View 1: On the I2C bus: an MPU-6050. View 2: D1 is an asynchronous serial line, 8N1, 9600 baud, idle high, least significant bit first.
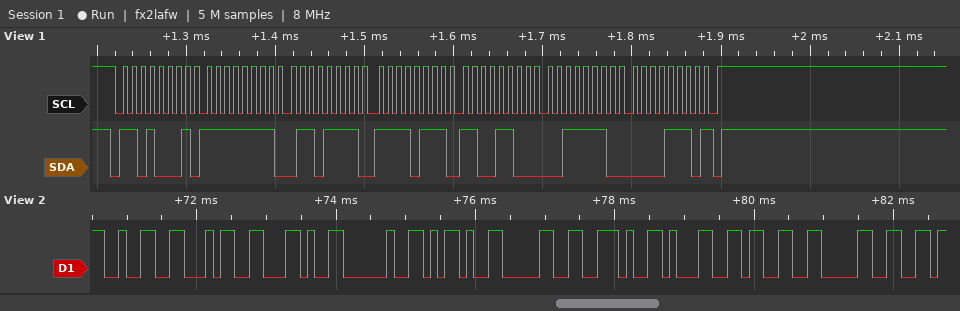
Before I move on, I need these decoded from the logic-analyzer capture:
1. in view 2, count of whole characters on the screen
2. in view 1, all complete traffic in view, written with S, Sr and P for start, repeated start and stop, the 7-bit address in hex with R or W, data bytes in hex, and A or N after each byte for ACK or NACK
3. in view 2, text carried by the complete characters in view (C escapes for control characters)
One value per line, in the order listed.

10
S 68R A FF A 6F A F7 A CC A 3E A 0E N P
"24, -0.130"
